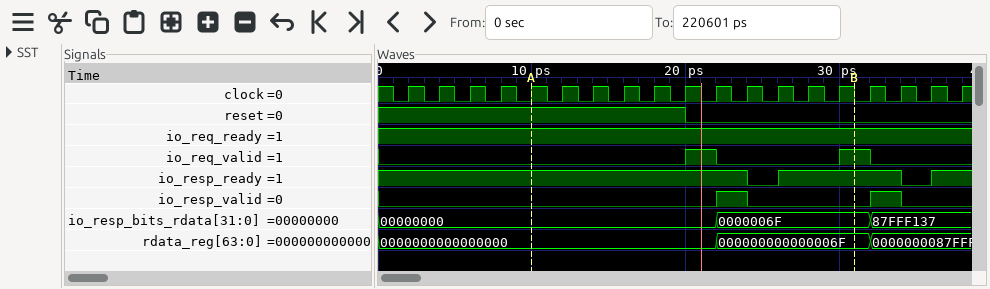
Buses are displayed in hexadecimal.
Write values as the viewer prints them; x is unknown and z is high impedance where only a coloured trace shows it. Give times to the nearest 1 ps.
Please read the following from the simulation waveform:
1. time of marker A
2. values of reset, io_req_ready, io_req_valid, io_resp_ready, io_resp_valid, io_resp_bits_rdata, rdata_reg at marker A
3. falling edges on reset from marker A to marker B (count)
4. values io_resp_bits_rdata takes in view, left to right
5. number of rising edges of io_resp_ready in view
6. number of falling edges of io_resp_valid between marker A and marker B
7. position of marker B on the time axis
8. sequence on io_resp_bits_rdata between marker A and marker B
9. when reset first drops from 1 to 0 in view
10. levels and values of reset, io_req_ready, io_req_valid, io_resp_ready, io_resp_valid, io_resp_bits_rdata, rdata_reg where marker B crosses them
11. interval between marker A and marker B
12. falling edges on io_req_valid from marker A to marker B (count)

10 ps
reset=1, io_req_ready=1, io_req_valid=0, io_resp_ready=1, io_resp_valid=0, io_resp_bits_rdata=00000000, rdata_reg=0000000000000000
1
00000000, 0000006F, 87FFF137
2
1
31 ps
00000000, 0000006F
20 ps
reset=0, io_req_ready=1, io_req_valid=1, io_resp_ready=1, io_resp_valid=0, io_resp_bits_rdata=0000006F, rdata_reg=000000000000006F
21 ps
1
